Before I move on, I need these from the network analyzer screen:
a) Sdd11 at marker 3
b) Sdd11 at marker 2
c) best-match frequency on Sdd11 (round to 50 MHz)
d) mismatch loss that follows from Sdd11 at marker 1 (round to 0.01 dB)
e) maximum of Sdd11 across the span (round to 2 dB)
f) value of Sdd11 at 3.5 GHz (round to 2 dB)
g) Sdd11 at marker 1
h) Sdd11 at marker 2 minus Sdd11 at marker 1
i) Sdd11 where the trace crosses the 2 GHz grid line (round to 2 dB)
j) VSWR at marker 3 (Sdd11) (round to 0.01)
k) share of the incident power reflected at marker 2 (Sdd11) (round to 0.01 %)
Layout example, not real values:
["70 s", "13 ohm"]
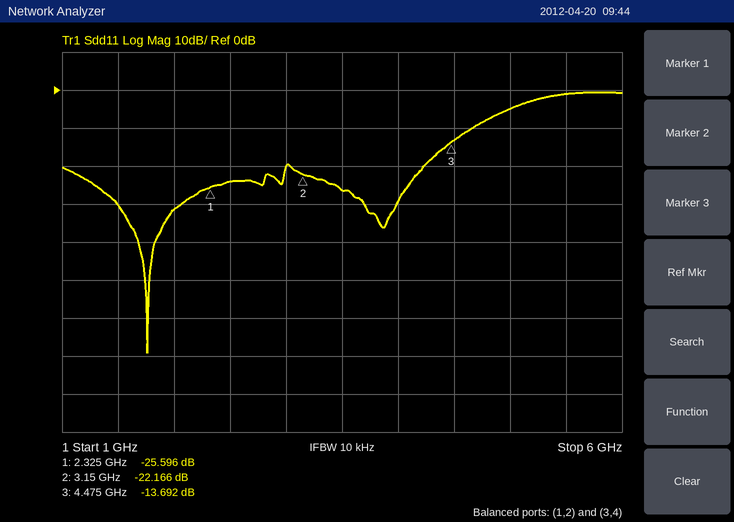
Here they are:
["-13.692 dB", "-22.166 dB", "1.75 GHz", "0.01 dB", "0 dB", "-26 dB", "-25.596 dB", "3.430 dB", "-32 dB", "1.52", "0.61 %"]
